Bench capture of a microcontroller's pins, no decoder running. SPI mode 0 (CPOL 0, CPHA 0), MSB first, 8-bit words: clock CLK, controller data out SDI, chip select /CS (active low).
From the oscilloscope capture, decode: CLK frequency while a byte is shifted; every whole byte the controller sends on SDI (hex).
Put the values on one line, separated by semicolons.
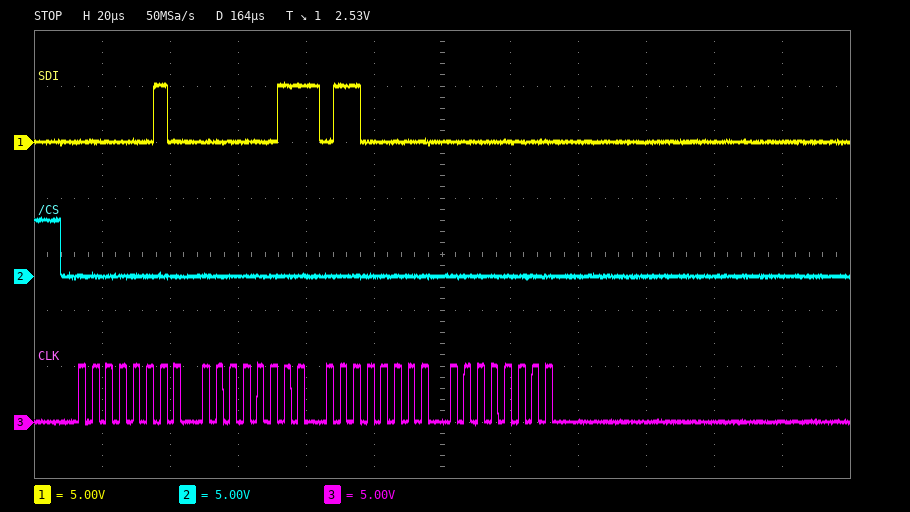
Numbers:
250 kHz; 02 03 60 00
